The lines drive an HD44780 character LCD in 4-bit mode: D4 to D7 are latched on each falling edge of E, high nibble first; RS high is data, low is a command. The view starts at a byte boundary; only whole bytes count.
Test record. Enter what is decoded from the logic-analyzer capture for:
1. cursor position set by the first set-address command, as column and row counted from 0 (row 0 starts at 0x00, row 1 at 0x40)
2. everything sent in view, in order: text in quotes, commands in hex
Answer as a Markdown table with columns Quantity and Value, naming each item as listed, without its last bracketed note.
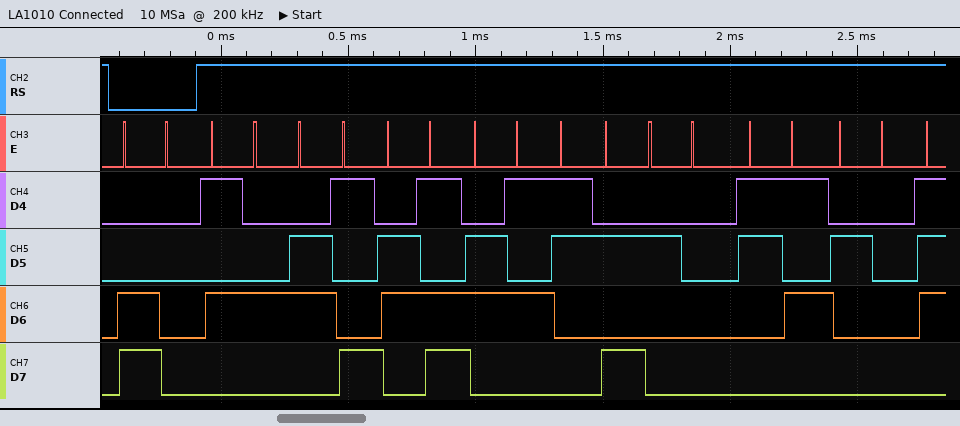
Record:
| Quantity | Value |
|---|---|
| cursor position set by the first set-address command, as column and row counted from 0 | column 0, row 1 |
| everything sent in view, in order: text in quotes, commands in hex | 0xC0 "Time: 5 " |
